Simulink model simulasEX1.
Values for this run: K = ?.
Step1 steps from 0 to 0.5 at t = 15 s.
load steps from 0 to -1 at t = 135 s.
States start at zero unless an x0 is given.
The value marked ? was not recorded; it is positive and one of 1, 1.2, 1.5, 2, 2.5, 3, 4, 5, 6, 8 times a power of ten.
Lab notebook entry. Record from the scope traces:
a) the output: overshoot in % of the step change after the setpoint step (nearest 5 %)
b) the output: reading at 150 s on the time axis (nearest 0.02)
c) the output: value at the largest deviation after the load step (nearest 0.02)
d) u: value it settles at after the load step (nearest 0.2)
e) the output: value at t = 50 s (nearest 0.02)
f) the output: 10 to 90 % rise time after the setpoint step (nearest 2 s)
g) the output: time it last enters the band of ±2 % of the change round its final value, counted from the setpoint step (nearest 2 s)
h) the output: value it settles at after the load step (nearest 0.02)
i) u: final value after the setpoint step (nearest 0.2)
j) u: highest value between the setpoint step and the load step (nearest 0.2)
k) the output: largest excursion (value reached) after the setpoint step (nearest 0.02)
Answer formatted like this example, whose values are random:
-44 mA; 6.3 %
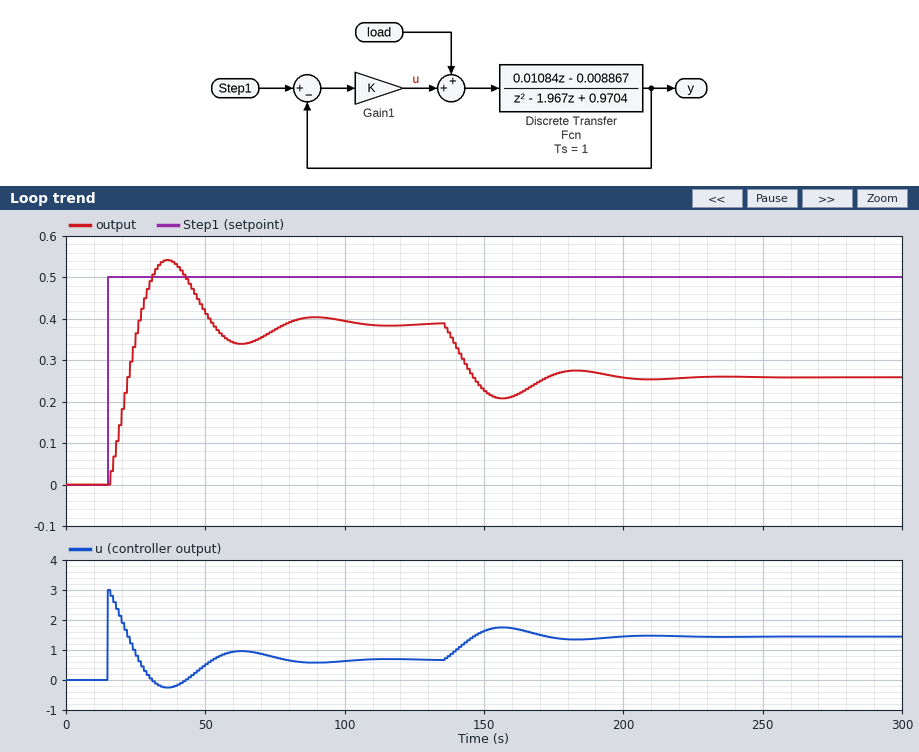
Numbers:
40 %; 0.22; 0.20; 1.4; 0.42; 8 s; 84 s; 0.26; 0.6; 3.0; 0.54
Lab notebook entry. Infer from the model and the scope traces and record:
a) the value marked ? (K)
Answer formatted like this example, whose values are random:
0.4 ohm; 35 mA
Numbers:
6
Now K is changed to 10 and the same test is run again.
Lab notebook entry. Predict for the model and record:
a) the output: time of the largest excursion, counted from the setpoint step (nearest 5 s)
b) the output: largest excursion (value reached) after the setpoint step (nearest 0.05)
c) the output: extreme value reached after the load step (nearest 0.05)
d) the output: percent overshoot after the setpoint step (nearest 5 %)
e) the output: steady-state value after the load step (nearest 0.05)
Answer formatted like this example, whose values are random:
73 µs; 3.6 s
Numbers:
15 s; 0.60; 0.30; 35 %; 0.35
